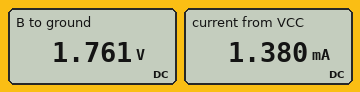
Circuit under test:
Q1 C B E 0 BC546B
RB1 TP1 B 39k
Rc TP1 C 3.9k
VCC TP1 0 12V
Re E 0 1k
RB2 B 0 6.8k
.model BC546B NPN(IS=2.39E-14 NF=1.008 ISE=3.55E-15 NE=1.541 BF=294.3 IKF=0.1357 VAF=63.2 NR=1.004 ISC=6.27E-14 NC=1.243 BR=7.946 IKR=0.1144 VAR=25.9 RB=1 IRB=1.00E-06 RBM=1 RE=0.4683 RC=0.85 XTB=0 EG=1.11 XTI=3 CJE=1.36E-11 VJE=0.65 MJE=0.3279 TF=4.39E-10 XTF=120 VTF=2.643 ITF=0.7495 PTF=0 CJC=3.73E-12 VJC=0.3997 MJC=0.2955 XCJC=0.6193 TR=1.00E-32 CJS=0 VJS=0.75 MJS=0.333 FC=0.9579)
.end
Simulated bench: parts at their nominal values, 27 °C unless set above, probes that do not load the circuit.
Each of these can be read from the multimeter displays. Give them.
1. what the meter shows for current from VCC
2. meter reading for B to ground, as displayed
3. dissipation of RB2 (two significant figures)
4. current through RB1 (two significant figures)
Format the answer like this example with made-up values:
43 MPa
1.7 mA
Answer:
1.380 mA
1.761 V
460 µW
260 µA
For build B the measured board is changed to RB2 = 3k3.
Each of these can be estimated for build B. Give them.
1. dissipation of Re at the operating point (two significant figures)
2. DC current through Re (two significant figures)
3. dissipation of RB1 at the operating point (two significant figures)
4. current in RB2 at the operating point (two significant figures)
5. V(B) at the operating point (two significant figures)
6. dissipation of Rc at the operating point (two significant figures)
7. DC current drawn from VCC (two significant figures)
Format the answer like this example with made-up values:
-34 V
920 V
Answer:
110 µW
330 µA
3.1 mW
280 µA
930 mV
420 µW
610 µA
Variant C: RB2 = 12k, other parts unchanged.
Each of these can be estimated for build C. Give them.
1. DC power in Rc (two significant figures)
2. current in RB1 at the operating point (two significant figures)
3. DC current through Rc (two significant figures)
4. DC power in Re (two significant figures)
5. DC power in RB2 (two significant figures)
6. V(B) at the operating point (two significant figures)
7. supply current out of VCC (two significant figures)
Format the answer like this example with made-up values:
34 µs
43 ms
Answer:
17 mW
240 µA
2.1 mA
4.4 mW
630 µW
2.8 V
2.3 mA
